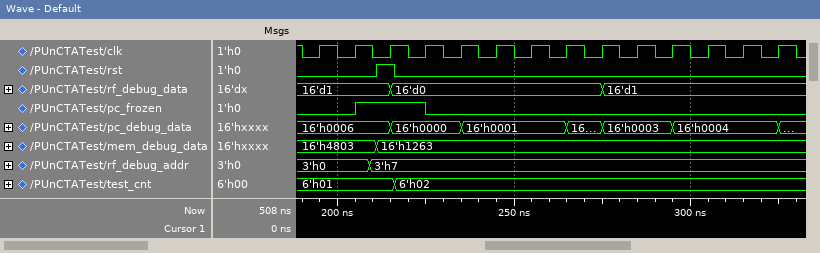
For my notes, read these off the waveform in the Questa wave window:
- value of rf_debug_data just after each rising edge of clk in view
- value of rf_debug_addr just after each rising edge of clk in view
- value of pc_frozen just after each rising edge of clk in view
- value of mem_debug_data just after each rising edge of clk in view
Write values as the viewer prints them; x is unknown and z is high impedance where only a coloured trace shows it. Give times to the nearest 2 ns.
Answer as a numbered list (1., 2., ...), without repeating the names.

1. 16'd1, 16'd1, 16'd0, 16'd0, 16'd0, 16'd0, 16'd0, 16'd0, 16'd1, 16'd1, 16'd1, 16'd1, 16'd1, 16'd1
2. 3'h0, 3'h0, 3'h7, 3'h7, 3'h7, 3'h7, 3'h7, 3'h7, 3'h7, 3'h7, 3'h7, 3'h7, 3'h7, 3'h7
3. 0 1 1 0 0 0 0 0 0 0 0 0 0 0
4. 16'h4803, 16'h4803, 16'h1263, 16'h1263, 16'h1263, 16'h1263, 16'h1263, 16'h1263, 16'h1263, 16'h1263, 16'h1263, 16'h1263, 16'h1263, 16'h1263
